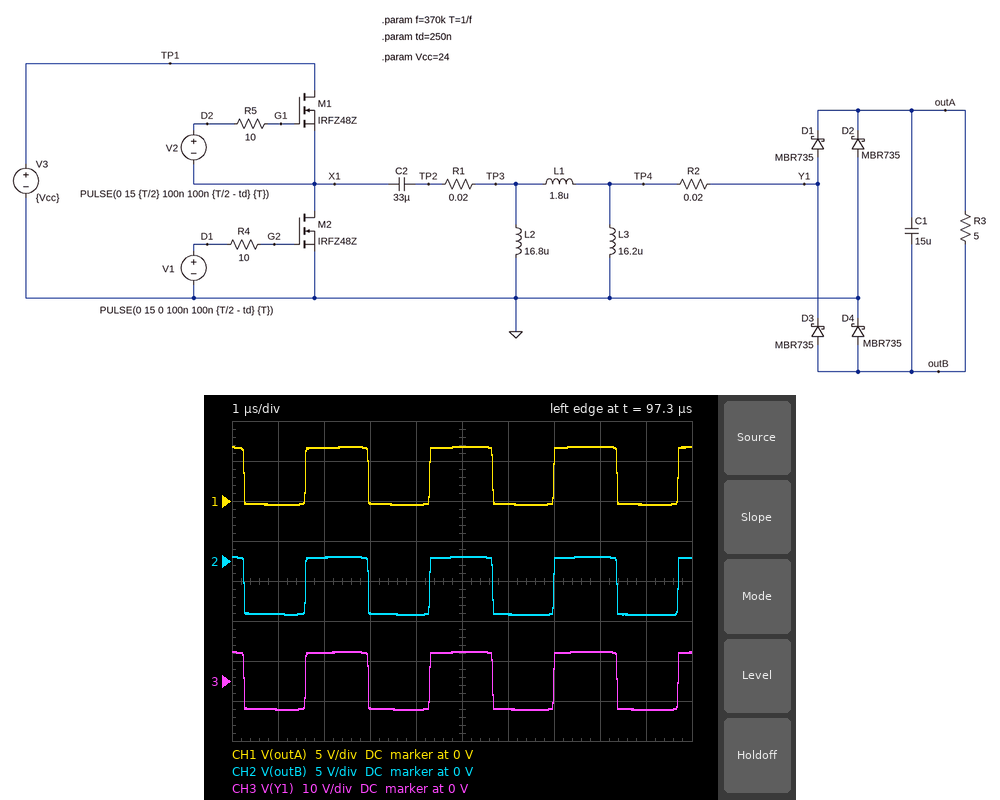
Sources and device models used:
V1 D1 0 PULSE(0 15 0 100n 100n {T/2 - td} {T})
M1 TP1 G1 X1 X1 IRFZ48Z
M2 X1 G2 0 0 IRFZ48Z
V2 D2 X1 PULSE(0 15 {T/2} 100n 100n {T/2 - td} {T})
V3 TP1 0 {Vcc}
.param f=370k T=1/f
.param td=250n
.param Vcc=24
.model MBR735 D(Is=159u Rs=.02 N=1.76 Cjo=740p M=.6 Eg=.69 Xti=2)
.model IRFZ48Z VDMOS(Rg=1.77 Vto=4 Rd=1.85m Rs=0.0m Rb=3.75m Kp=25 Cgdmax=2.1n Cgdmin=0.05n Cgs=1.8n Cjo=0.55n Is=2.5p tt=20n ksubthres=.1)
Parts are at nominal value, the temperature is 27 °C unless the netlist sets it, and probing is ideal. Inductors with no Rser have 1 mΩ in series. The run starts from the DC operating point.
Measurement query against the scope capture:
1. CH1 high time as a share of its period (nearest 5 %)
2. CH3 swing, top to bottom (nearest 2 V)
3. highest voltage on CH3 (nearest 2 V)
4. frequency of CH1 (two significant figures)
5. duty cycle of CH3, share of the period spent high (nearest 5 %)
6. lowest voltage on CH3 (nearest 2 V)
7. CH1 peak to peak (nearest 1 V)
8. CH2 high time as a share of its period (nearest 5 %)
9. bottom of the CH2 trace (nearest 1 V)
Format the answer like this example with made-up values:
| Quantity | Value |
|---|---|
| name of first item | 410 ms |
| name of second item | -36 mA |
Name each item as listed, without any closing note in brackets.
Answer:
| Quantity | Value |
|---|---|
| CH1 high time as a share of its period | 50 % |
| CH3 swing, top to bottom | 14 V |
| highest voltage on CH3 | 8 V |
| frequency of CH1 | 370 kHz |
| duty cycle of CH3, share of the period spent high | 50 % |
| lowest voltage on CH3 | -8 V |
| CH1 peak to peak | 7 V |
| CH2 high time as a share of its period | 50 % |
| bottom of the CH2 trace | -7 V |
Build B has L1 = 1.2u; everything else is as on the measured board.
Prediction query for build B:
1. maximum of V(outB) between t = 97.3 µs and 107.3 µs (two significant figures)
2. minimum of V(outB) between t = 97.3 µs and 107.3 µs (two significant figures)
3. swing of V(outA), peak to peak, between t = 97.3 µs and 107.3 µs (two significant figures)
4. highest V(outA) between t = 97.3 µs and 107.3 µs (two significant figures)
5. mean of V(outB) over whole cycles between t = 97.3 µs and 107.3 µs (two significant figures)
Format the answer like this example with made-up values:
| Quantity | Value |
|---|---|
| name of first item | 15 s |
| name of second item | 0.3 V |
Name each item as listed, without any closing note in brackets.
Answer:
| Quantity | Value |
|---|---|
| maximum of V(outB) between t = 97.3 µs and 107.3 µs | 510 mV |
| minimum of V(outB) between t = 97.3 µs and 107.3 µs | -8.2 V |
| swing of V(outA), peak to peak, between t = 97.3 µs and 107.3 µs | 8.7 V |
| highest V(outA) between t = 97.3 µs and 107.3 µs | 8.2 V |
| mean of V(outB) over whole cycles between t = 97.3 µs and 107.3 µs | -3.8 V |
